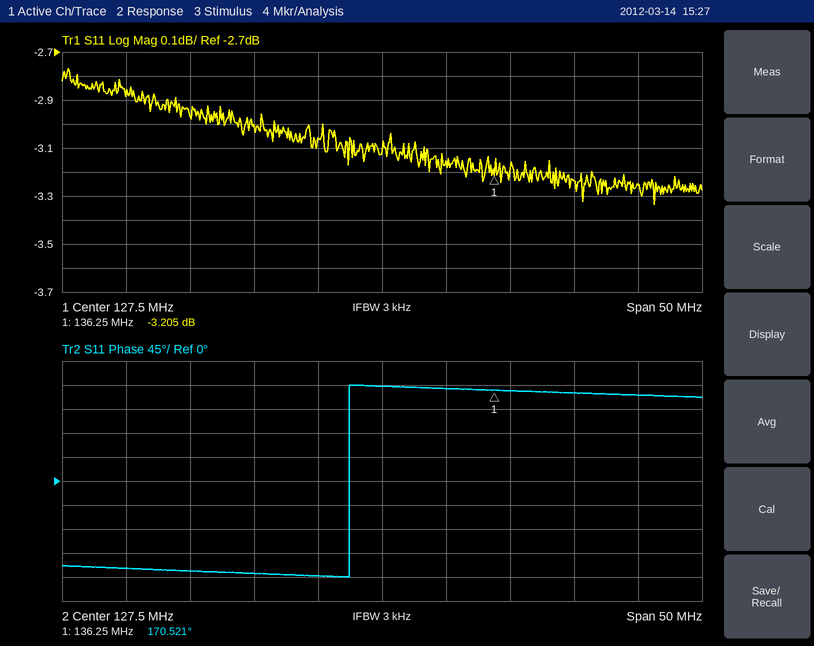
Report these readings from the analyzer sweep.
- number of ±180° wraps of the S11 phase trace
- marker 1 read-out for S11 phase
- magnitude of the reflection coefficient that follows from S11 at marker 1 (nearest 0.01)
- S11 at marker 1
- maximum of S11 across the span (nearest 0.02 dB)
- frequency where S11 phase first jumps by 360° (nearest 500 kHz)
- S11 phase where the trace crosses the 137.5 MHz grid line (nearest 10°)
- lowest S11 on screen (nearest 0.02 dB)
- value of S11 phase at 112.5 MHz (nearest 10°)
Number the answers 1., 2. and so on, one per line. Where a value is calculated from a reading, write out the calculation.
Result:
1. 1
2. 170.521°
3. 10^(-3.205/20) ≈ 0.69
4. -3.205 dB
5. -2.76 dB
6. 125.0 MHz
7. 170°
8. -3.34 dB
9. -170°
